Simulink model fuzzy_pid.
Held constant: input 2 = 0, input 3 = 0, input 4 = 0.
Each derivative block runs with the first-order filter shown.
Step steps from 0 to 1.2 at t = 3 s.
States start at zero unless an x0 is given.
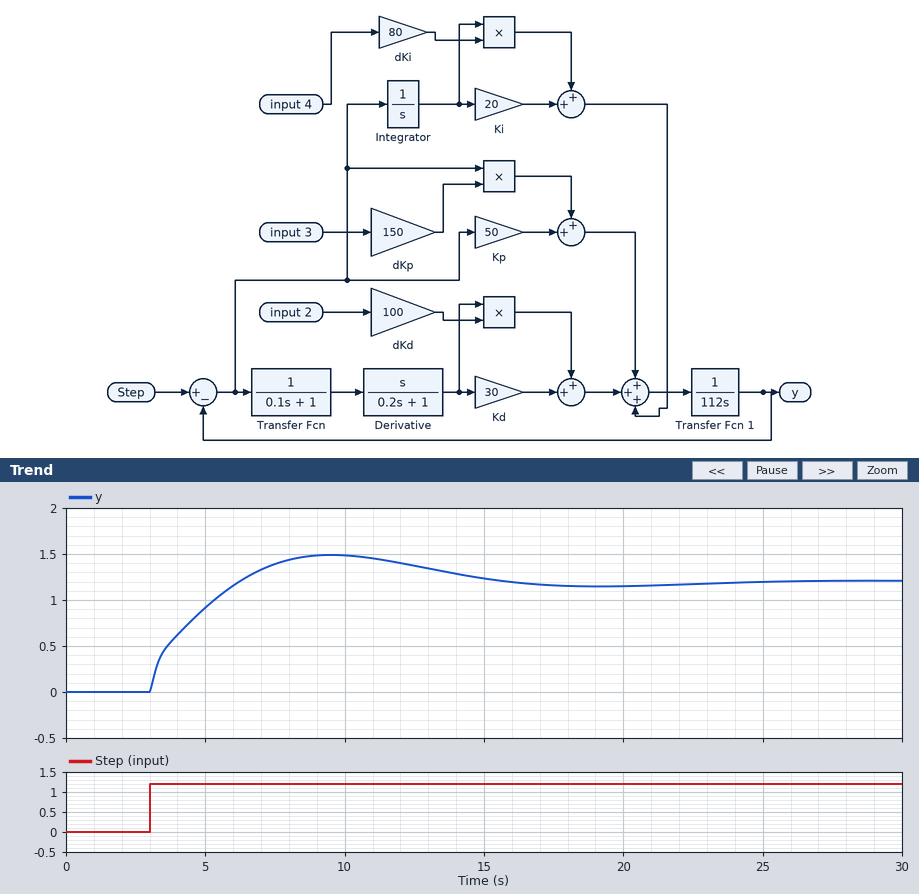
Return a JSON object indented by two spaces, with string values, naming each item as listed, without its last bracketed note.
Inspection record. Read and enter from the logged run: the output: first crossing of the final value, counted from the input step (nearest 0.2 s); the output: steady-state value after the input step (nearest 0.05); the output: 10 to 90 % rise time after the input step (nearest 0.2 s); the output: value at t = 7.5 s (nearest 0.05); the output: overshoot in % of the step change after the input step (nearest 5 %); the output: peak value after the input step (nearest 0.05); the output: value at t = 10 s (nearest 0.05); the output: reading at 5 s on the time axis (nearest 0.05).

{
  "the output: first crossing of the final value, counted from the input step": "3.2 s",
  "the output: steady-state value after the input step": "1.20",
  "the output: 10 to 90 % rise time after the input step": "2.6 s",
  "the output: value at t = 7.5 s": "1.40",
  "the output: overshoot in % of the step change after the input step": "25 %",
  "the output: peak value after the input step": "1.50",
  "the output: value at t = 10 s": "1.50",
  "the output: reading at 5 s on the time axis": "0.90"
}
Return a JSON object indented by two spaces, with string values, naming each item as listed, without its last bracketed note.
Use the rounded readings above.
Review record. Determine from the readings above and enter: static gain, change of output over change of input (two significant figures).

{
  "static gain, change of output over change of input": "1.0"
}
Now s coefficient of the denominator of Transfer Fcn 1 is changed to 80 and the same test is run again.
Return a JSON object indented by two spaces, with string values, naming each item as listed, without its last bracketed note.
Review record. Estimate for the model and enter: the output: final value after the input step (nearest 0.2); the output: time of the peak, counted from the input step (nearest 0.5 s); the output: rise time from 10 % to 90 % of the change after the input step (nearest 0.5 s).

{
  "the output: final value after the input step": "1.2",
  "the output: time of the peak, counted from the input step": "5.5 s",
  "the output: rise time from 10 % to 90 % of the change after the input step": "2.0 s"
}
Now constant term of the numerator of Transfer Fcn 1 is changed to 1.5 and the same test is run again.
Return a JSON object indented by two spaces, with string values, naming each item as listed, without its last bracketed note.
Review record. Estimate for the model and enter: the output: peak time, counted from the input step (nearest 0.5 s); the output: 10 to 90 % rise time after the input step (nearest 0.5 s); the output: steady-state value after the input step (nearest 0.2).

{
  "the output: peak time, counted from the input step": "5.5 s",
  "the output: 10 to 90 % rise time after the input step": "2.0 s",
  "the output: steady-state value after the input step": "1.2"
}
